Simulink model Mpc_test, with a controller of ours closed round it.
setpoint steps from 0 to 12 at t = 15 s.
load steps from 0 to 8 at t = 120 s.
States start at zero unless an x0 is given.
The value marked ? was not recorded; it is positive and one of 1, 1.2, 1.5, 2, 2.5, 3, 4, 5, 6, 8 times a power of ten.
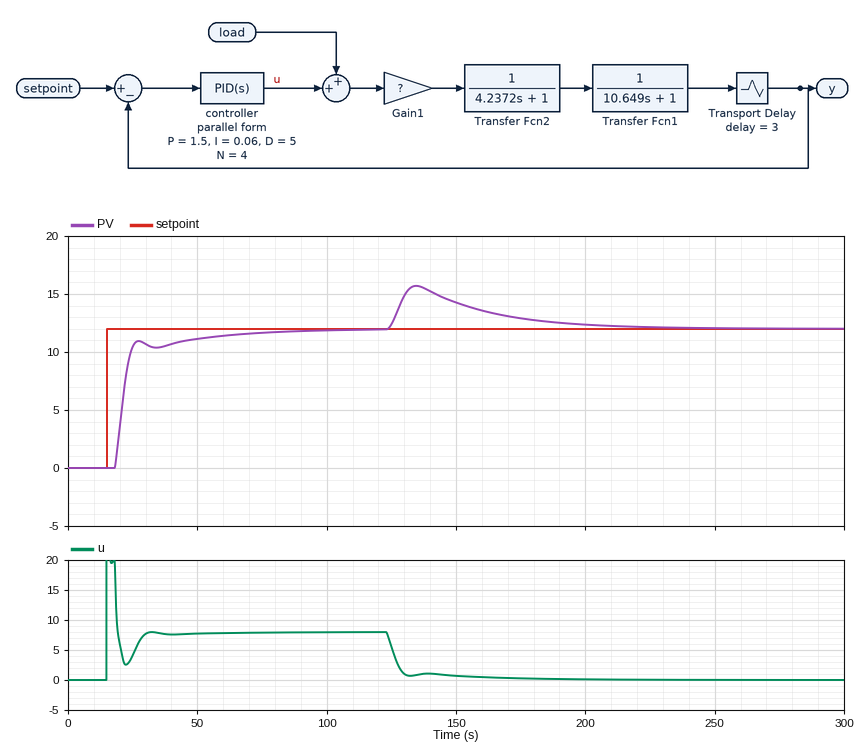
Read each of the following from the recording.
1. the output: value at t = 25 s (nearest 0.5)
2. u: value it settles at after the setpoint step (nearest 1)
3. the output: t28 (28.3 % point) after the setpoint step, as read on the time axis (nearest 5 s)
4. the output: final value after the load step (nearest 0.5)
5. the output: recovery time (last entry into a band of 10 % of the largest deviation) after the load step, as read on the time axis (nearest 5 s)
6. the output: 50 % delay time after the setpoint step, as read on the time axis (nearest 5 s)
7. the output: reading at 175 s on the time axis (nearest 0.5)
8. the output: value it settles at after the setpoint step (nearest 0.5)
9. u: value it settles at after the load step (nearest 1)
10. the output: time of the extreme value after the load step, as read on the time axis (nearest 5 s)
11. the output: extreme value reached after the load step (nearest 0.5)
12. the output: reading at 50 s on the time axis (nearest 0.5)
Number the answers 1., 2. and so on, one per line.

1. 10.5
2. 8
3. 20 s
4. 12.0
5. 200 s
6. 20 s
7. 13.0
8. 12.0
9. 0
10. 135 s
11. 15.5
12. 11.0
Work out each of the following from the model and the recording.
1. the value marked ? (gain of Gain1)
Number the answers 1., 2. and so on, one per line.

1. 1.5
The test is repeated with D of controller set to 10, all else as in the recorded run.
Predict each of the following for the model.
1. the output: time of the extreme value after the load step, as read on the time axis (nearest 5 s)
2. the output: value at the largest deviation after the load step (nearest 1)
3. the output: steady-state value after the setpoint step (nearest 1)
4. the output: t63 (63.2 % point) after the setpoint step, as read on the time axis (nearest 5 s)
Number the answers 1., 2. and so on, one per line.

1. 140 s
2. 15
3. 12
4. 20 s
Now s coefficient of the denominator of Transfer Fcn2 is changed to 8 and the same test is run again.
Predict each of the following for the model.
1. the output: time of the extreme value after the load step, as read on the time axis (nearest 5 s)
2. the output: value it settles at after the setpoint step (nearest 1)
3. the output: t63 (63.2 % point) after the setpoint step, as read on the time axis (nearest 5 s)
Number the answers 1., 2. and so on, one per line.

1. 140 s
2. 12
3. 25 s
